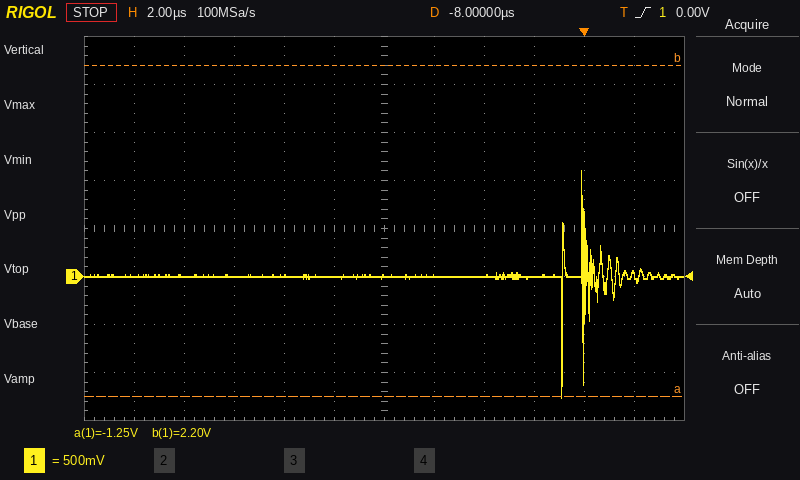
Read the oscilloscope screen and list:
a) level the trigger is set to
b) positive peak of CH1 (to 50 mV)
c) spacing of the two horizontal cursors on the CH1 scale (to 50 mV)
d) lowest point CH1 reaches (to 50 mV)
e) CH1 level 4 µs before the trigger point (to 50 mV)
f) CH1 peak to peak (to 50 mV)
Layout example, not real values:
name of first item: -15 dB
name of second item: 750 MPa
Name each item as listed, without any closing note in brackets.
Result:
level the trigger is set to: 0.00 V
positive peak of CH1: 1.10 V
spacing of the two horizontal cursors on the CH1 scale: 3.45 V
lowest point CH1 reaches: -1.25 V
CH1 level 4 µs before the trigger point: 0 mV
CH1 peak to peak: 2.35 V
